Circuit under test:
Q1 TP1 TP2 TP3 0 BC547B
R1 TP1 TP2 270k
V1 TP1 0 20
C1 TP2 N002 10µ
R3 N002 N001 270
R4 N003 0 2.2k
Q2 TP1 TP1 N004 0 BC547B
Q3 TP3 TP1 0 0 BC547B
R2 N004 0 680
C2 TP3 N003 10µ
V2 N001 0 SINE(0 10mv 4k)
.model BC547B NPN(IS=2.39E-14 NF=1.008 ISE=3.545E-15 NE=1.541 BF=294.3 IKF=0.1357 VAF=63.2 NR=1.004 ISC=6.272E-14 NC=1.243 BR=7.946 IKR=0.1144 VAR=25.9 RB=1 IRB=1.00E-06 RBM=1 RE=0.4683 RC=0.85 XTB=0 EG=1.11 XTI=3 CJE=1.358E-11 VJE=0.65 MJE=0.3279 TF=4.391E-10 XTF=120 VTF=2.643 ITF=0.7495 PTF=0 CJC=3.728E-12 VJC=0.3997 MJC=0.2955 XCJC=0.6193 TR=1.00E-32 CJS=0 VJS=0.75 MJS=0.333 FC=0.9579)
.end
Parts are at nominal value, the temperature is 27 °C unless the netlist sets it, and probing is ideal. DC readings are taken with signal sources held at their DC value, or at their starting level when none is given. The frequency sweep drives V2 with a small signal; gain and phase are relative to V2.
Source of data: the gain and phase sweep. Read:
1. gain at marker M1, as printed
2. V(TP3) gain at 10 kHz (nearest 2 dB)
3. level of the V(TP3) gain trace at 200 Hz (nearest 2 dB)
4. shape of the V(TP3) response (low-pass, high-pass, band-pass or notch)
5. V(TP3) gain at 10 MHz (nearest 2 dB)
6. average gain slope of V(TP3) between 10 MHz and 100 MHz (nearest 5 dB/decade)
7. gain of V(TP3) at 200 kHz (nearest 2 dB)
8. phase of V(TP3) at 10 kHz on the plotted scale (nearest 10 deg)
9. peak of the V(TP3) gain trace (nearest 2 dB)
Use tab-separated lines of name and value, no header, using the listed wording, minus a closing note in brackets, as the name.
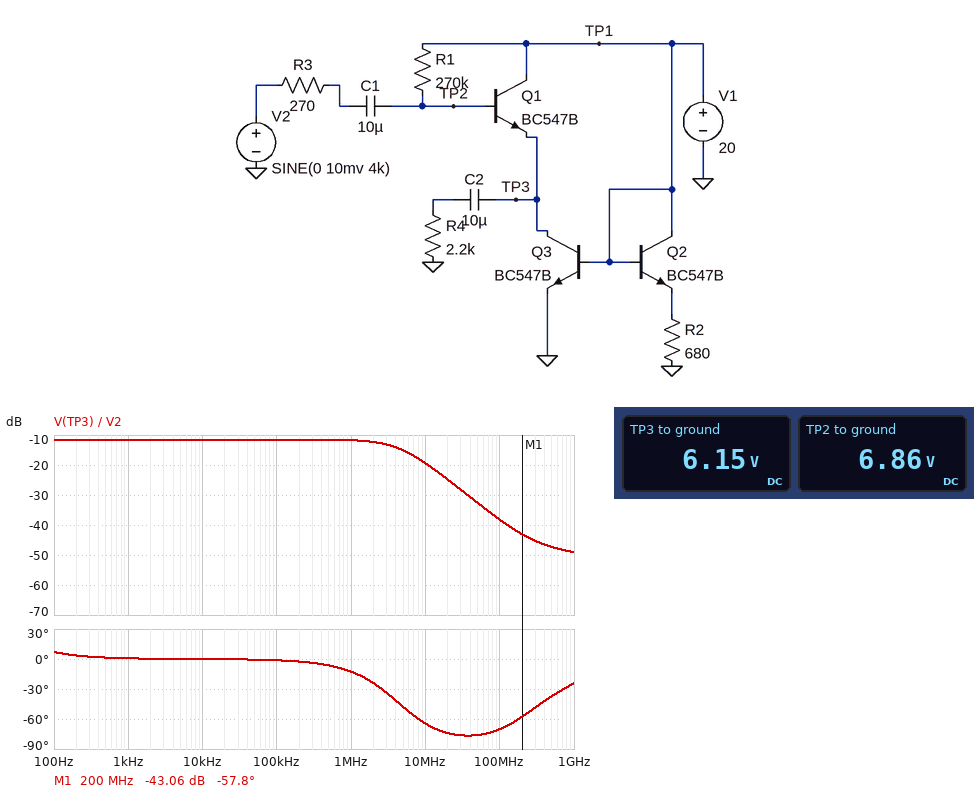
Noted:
gain at marker M1, as printed	-43.06 dB
V(TP3) gain at 10 kHz	-12 dB
level of the V(TP3) gain trace at 200 Hz	-12 dB
shape of the V(TP3) response	low-pass
V(TP3) gain at 10 MHz	-20 dB
average gain slope of V(TP3) between 10 MHz and 100 MHz	-20 dB/decade
gain of V(TP3) at 200 kHz	-12 dB
phase of V(TP3) at 10 kHz on the plotted scale	0 deg
peak of the V(TP3) gain trace	-12 dB
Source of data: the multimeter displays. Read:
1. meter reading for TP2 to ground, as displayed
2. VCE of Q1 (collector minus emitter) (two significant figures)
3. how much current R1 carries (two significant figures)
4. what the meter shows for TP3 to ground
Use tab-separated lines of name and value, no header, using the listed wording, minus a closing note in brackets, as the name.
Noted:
meter reading for TP2 to ground, as displayed	6.86 V
VCE of Q1 (collector minus emitter)	14 V
how much current R1 carries	49 µA
what the meter shows for TP3 to ground	6.15 V
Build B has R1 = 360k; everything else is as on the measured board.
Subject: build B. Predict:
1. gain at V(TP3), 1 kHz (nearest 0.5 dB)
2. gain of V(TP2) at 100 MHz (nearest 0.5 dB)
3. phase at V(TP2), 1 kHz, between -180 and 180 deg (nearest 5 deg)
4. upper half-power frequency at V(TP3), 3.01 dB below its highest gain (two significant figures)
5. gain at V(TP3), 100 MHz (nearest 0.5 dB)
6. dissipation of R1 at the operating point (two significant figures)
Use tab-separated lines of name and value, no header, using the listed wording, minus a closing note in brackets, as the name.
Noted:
gain at V(TP3), 1 kHz	-12.5 dB
gain of V(TP2) at 100 MHz	-28.0 dB
phase at V(TP2), 1 kHz, between -180 and 180 deg	0 deg
upper half-power frequency at V(TP3), 3.01 dB below its highest gain	4.6 MHz
gain at V(TP3), 100 MHz	-38.5 dB
dissipation of R1 at the operating point	480 µW
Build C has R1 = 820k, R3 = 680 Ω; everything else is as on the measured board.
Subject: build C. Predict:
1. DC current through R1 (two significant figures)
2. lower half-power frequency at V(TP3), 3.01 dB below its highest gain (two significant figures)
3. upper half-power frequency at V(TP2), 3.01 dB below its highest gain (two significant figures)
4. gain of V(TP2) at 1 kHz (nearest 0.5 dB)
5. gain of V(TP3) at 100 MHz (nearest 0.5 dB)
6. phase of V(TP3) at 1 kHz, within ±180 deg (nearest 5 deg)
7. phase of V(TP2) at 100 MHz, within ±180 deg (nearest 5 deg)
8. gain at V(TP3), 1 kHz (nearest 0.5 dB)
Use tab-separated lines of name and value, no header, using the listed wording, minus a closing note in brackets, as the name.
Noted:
DC current through R1	16 µA
lower half-power frequency at V(TP3), 3.01 dB below its highest gain	5.6 Hz
upper half-power frequency at V(TP2), 3.01 dB below its highest gain	2.7 MHz
gain of V(TP2) at 1 kHz	-2.5 dB
gain of V(TP3) at 100 MHz	-48.0 dB
phase of V(TP3) at 1 kHz, within ±180 deg	0 deg
phase of V(TP2) at 100 MHz, within ±180 deg	-80 deg
gain at V(TP3), 1 kHz	-17.5 dB
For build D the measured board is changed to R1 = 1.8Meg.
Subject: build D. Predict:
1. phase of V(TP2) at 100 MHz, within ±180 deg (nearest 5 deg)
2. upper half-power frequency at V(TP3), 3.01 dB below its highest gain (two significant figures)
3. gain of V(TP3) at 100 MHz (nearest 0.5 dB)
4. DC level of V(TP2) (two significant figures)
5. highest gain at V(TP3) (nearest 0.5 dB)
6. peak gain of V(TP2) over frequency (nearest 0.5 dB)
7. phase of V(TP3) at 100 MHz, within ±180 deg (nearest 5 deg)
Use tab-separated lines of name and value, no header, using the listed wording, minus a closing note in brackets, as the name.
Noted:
phase of V(TP2) at 100 MHz, within ±180 deg	-80 deg
upper half-power frequency at V(TP3), 3.01 dB below its highest gain	7.4 MHz
gain of V(TP3) at 100 MHz	-42.0 dB
DC level of V(TP2)	6.8 V
highest gain at V(TP3)	-21.0 dB
peak gain of V(TP2) over frequency	-0.5 dB
phase of V(TP3) at 100 MHz, within ±180 deg	-55 deg
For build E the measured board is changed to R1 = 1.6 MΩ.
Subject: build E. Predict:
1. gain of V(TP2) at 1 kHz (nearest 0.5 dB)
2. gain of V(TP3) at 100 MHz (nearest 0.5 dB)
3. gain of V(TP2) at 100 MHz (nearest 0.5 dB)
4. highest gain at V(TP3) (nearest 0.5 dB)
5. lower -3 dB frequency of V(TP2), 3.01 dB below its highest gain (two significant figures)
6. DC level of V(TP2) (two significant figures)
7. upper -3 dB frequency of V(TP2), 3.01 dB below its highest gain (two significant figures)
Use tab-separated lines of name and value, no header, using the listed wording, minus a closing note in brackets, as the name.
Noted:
gain of V(TP2) at 1 kHz	-0.5 dB
gain of V(TP3) at 100 MHz	-42.0 dB
gain of V(TP2) at 100 MHz	-23.5 dB
highest gain at V(TP3)	-20.0 dB
lower -3 dB frequency of V(TP2), 3.01 dB below its highest gain	4.0 Hz
DC level of V(TP2)	6.8 V
upper -3 dB frequency of V(TP2), 3.01 dB below its highest gain	7.1 MHz
